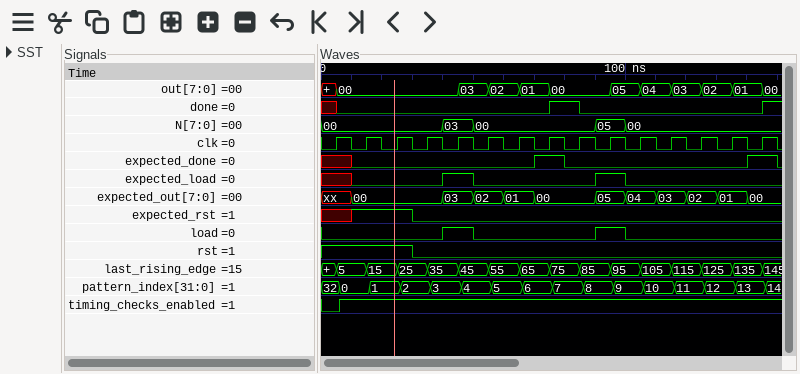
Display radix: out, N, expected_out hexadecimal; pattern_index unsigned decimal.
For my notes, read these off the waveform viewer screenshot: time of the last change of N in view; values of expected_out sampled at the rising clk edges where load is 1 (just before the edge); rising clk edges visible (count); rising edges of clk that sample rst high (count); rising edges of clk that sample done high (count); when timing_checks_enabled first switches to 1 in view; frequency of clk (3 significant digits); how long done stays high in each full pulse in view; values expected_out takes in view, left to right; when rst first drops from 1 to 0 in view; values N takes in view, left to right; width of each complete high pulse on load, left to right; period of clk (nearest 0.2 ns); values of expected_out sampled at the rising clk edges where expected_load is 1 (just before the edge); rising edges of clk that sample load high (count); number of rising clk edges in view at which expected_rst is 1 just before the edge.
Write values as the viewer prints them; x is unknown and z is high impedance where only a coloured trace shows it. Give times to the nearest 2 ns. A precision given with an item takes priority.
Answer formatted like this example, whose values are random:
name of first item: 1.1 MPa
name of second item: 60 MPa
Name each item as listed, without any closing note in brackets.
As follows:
time of the last change of N in view: 100 ns
values of expected_out sampled at the rising clk edges where load is 1: 03, 05
rising clk edges visible: 15
rising edges of clk that sample rst high: 3
rising edges of clk that sample done high: 1
when timing_checks_enabled first switches to 1 in view: 6 ns
frequency of clk: 100 MHz
how long done stays high in each full pulse in view: 10 ns
values expected_out takes in view, left to right: xx, 00, 03, 02, 01, 00, 05, 04, 03, 02, 01, 00
when rst first drops from 1 to 0 in view: 30 ns
values N takes in view, left to right: 00, 03, 00, 05, 00
width of each complete high pulse on load, left to right: 10 ns, 10 ns
period of clk: 10 ns
values of expected_out sampled at the rising clk edges where expected_load is 1: 03, 05
rising edges of clk that sample load high: 2
number of rising clk edges in view at which expected_rst is 1 just before the edge: 2
